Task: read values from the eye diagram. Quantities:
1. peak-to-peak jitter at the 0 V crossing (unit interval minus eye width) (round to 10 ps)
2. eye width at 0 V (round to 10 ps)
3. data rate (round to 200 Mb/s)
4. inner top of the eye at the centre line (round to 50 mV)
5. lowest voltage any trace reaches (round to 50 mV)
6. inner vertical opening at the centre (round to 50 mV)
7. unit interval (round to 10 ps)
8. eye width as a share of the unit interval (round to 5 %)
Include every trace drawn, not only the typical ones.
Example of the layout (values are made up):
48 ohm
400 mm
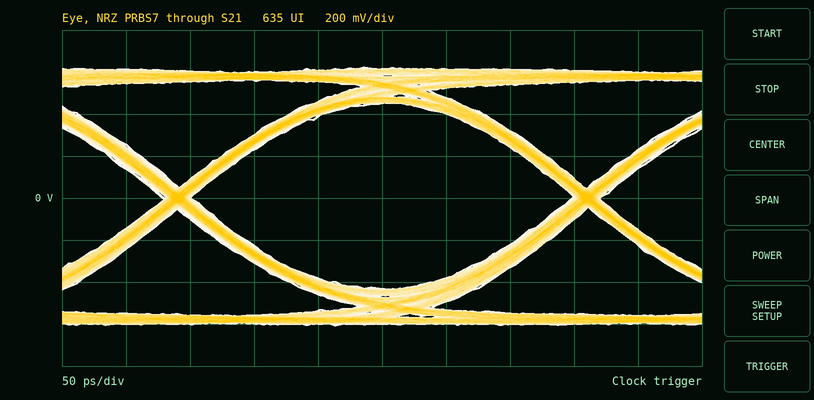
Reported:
20 ps
300 ps
3.2 Gb/s
450 mV
-600 mV
900 mV
320 ps
95 %
